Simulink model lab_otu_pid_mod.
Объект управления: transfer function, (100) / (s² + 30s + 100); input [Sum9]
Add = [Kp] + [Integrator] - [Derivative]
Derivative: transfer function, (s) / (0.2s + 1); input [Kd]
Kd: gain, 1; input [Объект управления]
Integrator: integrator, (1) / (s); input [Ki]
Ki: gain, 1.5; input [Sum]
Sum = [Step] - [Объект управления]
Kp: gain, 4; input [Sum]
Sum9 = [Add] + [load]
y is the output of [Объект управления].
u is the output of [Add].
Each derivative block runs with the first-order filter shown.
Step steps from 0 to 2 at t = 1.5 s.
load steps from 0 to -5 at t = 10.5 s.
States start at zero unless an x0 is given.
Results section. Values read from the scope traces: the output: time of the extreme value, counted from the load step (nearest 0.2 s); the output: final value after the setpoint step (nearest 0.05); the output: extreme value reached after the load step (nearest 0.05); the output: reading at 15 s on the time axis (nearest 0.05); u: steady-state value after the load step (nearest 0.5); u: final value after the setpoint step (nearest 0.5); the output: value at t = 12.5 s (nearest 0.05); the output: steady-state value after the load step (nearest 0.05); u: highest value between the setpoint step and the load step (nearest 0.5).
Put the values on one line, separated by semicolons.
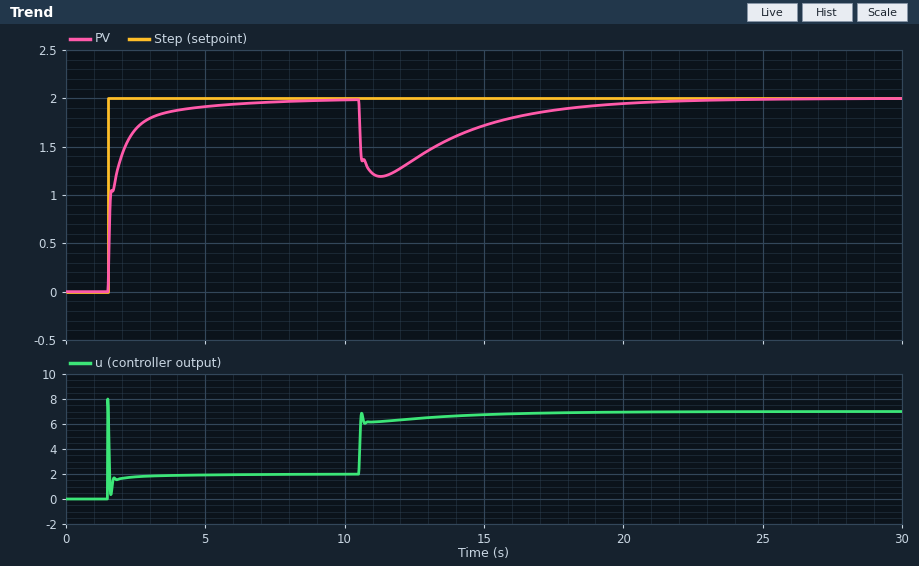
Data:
0.8 s; 2.00; 1.20; 1.70; 7.0; 2.0; 1.35; 2.00; 8.0
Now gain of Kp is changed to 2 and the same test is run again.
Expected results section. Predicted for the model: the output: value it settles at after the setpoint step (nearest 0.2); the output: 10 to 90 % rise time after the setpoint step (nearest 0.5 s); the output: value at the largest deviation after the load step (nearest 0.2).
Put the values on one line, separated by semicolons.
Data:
2.0; 1.5 s; 0.8
